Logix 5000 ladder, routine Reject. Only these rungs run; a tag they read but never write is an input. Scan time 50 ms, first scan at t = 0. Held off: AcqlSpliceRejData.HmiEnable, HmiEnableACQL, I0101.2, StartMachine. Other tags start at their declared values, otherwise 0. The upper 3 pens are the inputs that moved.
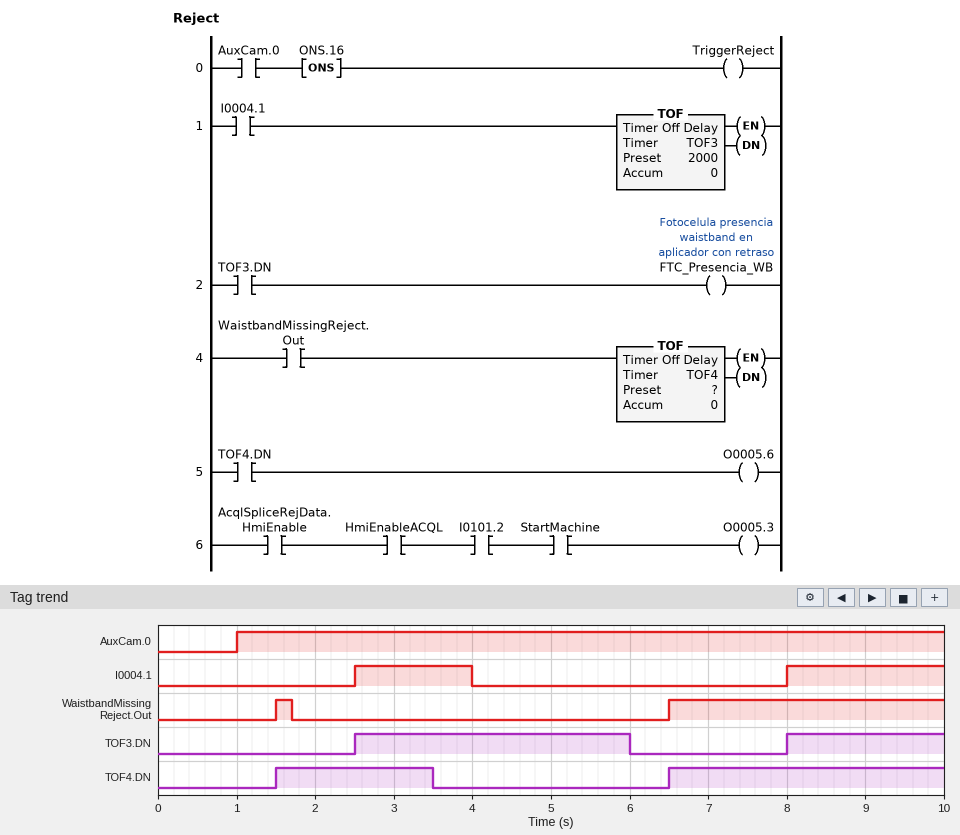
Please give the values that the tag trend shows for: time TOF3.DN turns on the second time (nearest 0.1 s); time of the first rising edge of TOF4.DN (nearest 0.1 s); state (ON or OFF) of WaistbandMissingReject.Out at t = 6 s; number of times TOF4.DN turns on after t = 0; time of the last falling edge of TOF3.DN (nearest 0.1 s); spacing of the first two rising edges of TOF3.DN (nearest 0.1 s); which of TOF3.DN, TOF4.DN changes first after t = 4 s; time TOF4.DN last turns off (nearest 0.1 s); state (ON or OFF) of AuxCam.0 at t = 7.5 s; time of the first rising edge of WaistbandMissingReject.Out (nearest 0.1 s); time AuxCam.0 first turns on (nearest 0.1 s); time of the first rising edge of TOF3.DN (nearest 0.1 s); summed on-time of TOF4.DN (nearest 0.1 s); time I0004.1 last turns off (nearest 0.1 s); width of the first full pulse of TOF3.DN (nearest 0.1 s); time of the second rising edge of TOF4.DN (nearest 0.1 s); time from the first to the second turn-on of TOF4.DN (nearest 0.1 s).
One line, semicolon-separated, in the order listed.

8.0 s; 1.5 s; OFF; 2; 6.0 s; 5.5 s; TOF3.DN; 3.5 s; ON; 1.5 s; 1.0 s; 2.5 s; 5.5 s; 4.0 s; 3.5 s; 6.5 s; 5.0 s
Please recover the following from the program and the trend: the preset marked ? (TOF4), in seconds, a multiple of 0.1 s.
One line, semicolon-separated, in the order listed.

1.8 s
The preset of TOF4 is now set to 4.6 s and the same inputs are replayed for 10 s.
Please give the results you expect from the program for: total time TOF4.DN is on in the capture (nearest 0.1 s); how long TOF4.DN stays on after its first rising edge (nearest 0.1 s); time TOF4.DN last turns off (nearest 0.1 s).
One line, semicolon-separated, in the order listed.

8.3 s; 4.8 s; 6.3 s
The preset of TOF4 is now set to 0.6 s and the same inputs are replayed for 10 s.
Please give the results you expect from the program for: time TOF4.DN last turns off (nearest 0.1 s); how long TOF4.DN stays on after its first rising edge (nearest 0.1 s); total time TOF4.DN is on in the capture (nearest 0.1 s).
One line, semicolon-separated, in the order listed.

2.3 s; 0.8 s; 4.3 s
